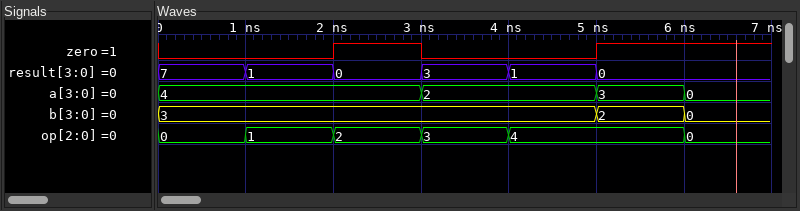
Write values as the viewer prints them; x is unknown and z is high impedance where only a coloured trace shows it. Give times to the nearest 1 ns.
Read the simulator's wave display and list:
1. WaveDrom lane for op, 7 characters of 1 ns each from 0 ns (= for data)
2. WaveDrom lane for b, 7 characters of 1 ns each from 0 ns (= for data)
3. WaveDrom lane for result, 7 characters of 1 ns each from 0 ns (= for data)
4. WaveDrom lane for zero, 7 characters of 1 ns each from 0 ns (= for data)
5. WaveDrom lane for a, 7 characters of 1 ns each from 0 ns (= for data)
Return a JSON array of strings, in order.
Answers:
["{name: 'op', wave: '=====.=', data: '0 1 2 3 4 0'}", "{name: 'b', wave: '=....==', data: '3 2 0'}", "{name: 'result', wave: '======.', data: '7 1 0 3 1 0'}", "{name: 'zero', wave: '0.10.1.'}", "{name: 'a', wave: '=..=.==', data: '4 2 3 0'}"]
